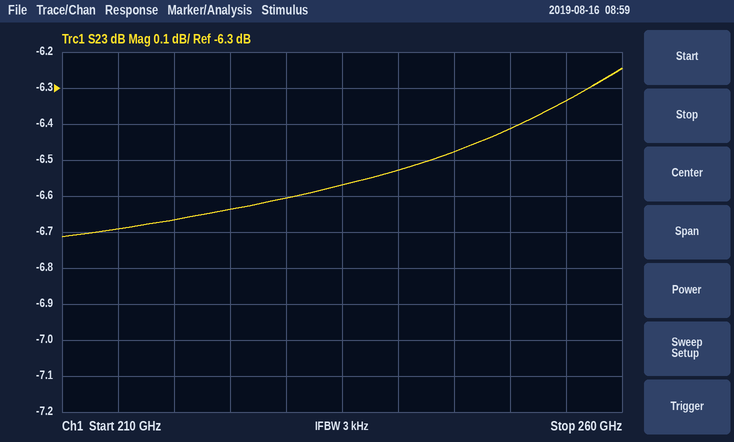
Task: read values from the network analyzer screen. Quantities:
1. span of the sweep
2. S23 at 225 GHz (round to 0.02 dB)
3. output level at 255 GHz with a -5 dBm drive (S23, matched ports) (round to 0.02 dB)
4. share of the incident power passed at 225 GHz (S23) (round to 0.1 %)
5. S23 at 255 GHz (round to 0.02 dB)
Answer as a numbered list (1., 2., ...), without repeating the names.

1. 50 GHz
2. -6.64 dB
3. -11.34 dBm
4. 21.7 %
5. -6.34 dB
